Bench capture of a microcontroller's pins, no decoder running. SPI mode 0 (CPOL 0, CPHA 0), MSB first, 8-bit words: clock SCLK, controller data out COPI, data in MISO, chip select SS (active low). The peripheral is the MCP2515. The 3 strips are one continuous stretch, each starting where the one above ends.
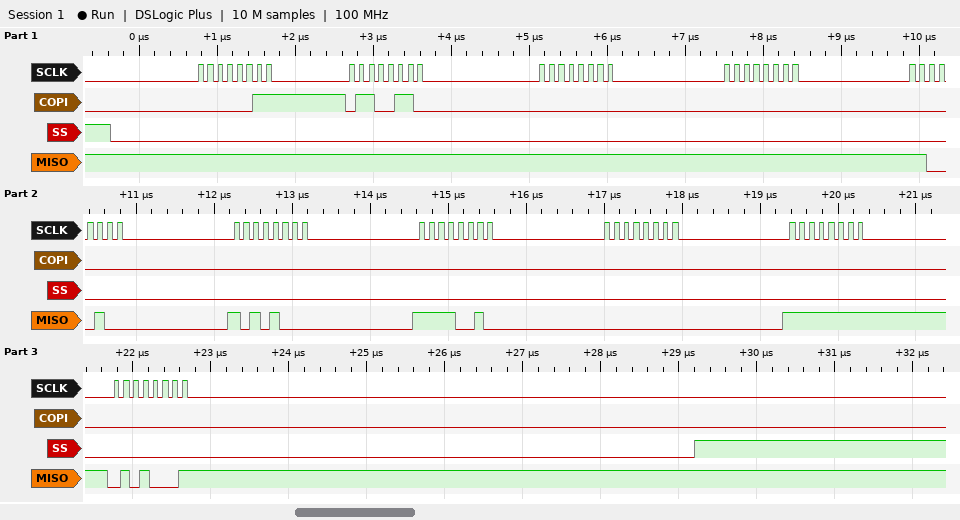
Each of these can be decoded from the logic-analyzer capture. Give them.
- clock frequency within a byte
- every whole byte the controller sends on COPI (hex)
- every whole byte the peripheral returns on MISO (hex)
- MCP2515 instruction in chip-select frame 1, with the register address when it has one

8 MHz
03 66 00 00 00 00 00 00 00 00
FF FF FF FF C4 A8 F2 00 FF 51
READ 0x66
